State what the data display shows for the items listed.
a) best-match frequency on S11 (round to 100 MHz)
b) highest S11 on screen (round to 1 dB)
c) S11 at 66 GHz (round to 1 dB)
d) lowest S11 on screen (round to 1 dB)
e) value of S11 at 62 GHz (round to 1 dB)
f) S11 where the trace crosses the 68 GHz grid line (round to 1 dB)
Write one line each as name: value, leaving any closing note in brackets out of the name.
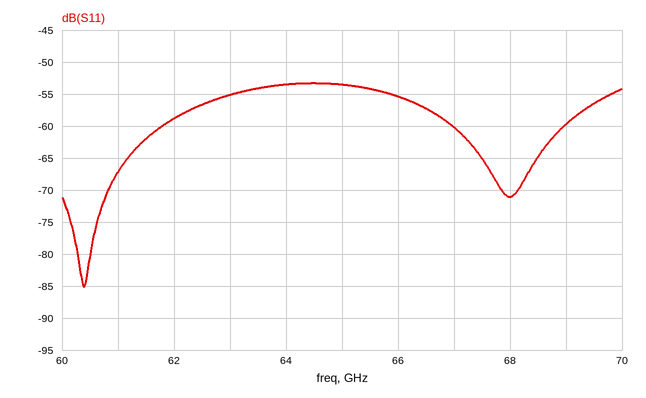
best-match frequency on S11: 60.4 GHz
highest S11 on screen: -53 dB
S11 at 66 GHz: -55 dB
lowest S11 on screen: -85 dB
value of S11 at 62 GHz: -59 dB
S11 where the trace crosses the 68 GHz grid line: -71 dB
